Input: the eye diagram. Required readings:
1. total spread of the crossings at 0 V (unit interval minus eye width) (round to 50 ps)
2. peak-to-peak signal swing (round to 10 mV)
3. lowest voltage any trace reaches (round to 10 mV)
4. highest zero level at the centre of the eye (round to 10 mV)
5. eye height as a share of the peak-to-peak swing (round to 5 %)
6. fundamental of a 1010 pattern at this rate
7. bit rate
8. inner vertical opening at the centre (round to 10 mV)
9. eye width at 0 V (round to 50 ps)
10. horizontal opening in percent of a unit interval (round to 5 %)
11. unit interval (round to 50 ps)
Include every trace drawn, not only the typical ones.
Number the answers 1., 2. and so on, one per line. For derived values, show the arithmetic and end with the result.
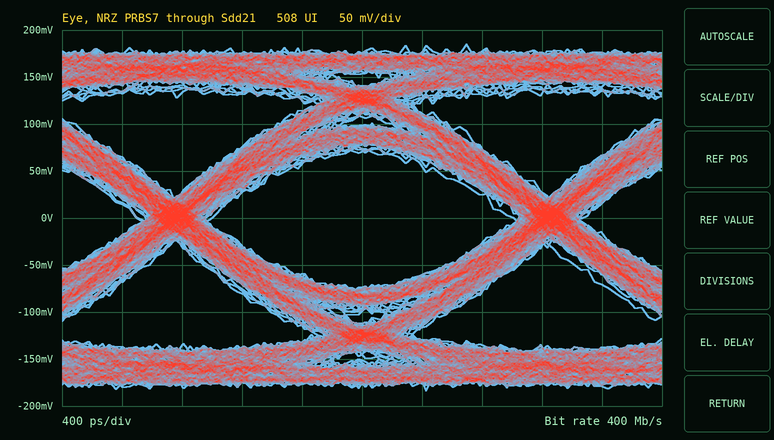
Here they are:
1. 500 ps
2. 370 mV
3. -180 mV
4. -70 mV
5. 140 mV / 370 mV ≈ 37.8 %, so 40 % to the nearest 5 %
6. 200 MHz
7. 400 Mb/s
8. 140 mV
9. 2.00 ns
10. 2.00 ns / 2.50 ns ≈ 80 %
11. 2.50 ns
